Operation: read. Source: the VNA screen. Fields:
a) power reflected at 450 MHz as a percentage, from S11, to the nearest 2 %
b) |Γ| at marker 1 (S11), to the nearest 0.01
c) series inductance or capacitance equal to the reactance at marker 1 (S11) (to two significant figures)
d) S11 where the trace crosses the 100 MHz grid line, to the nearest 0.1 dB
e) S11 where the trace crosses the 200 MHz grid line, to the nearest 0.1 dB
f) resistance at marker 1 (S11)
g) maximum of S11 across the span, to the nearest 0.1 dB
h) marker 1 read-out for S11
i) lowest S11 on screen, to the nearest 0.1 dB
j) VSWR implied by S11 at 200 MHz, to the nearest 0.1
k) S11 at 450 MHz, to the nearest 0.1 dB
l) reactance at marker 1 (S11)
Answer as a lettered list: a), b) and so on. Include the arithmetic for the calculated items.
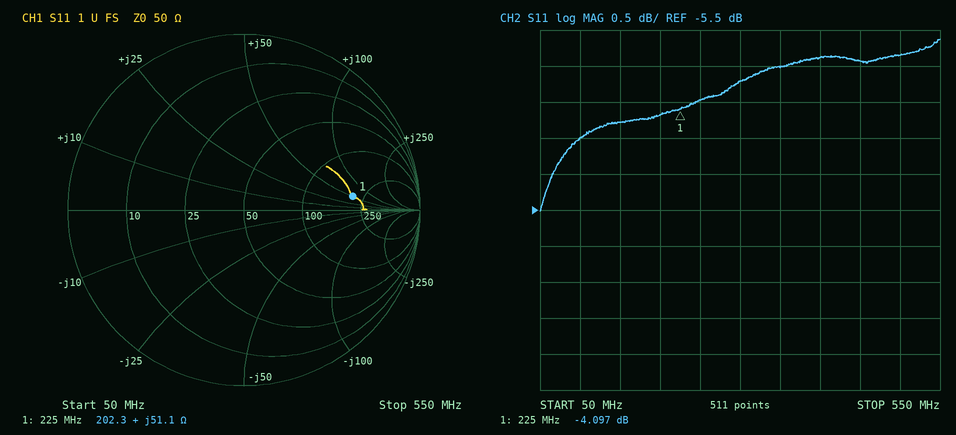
a) 10^(-3.4/10) ≈ 46 %
b) 0.62
c) L = 51.1 Ω/(2π × 225 MHz) ≈ 36 nH
d) -4.5 dB
e) -4.2 dB
f) 202.3 Ω
g) -3.1 dB
h) -4.097 dB
i) -5.5 dB
j) |Γ| = 10^(-4.2/20) = 0.6166; VSWR = (1 + 0.6166)/(1 − 0.6166) ≈ 4.2
k) -3.4 dB
l) +51.1 Ω
